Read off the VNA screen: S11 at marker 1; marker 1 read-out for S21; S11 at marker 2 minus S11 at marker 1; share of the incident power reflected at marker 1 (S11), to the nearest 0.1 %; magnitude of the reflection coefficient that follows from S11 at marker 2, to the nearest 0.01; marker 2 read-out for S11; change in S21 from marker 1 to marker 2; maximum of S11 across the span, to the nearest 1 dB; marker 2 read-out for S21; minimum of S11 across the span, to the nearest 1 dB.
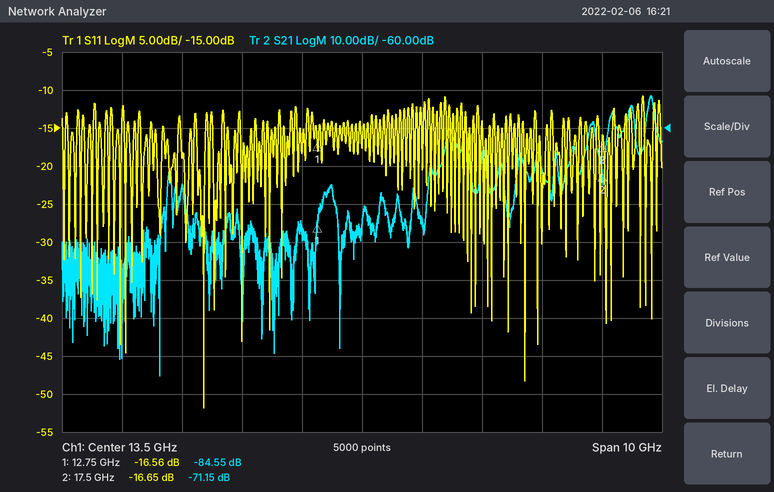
-16.56 dB
-84.55 dB
-0.09 dB
2.2 %
0.15
-16.65 dB
13.40 dB
-11 dB
-71.15 dB
-52 dB
